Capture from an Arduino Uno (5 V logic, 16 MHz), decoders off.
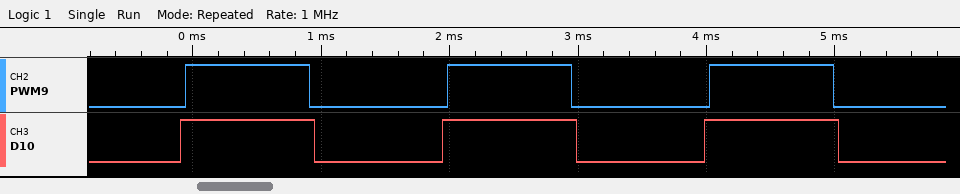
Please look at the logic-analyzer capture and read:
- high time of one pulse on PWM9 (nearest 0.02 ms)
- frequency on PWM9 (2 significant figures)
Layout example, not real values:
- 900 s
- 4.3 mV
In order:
- 0.96 ms
- 490 Hz
